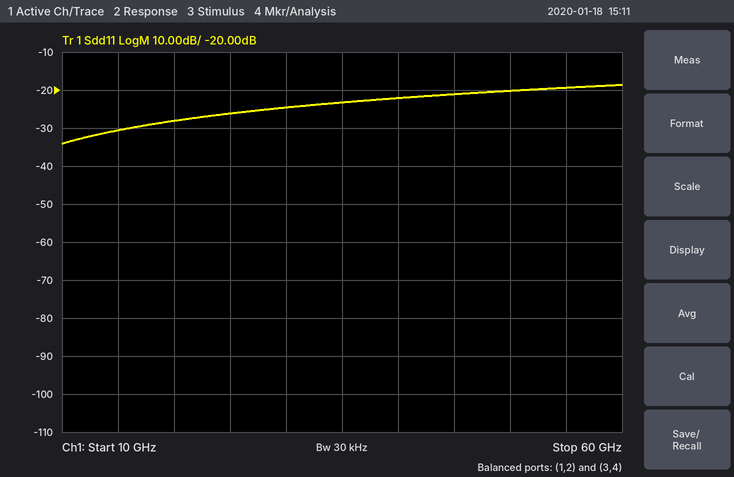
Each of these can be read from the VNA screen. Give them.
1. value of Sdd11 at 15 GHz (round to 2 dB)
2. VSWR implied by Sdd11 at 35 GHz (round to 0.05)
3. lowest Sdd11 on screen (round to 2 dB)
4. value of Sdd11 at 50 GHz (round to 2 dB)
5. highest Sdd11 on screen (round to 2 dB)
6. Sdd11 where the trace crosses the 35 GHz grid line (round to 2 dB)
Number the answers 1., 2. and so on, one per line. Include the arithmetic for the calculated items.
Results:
1. -30 dB
2. |Γ| = 10^(-24/20) = 0.0631; VSWR = (1 + 0.0631)/(1 − 0.0631) ≈ 1.13, so 1.15 to the nearest 0.05
3. -34 dB
4. -20 dB
5. -18 dB
6. -24 dB
